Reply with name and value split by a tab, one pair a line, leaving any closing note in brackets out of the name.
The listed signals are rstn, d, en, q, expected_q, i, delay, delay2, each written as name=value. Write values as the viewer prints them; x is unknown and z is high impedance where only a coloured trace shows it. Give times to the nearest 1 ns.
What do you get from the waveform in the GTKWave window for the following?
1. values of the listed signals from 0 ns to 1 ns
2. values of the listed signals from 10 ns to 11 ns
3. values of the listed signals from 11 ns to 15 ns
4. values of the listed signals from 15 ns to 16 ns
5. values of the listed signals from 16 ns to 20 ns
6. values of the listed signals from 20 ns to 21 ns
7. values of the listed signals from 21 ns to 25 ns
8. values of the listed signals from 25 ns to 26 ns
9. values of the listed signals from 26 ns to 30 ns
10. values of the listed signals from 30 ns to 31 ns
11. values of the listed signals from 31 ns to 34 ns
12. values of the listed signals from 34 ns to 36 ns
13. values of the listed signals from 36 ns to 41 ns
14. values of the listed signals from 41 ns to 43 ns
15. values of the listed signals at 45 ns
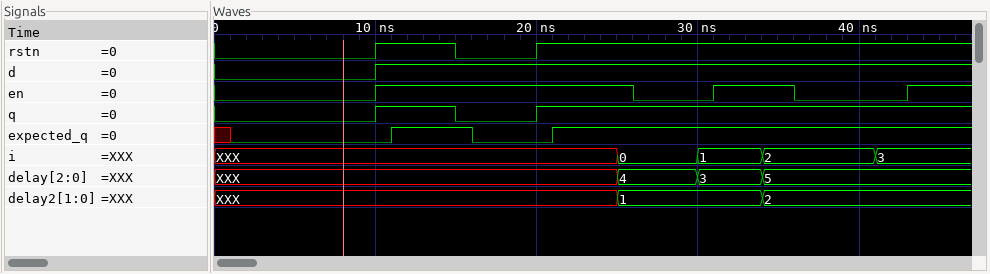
values of the listed signals from 0 ns to 1 ns	rstn=0, d=0, en=0, q=0, expected_q=x, i=XXX, delay=XXX, delay2=XXX
values of the listed signals from 10 ns to 11 ns	rstn=1, d=1, en=1, q=1, expected_q=0, i=XXX, delay=XXX, delay2=XXX
values of the listed signals from 11 ns to 15 ns	rstn=1, d=1, en=1, q=1, expected_q=1, i=XXX, delay=XXX, delay2=XXX
values of the listed signals from 15 ns to 16 ns	rstn=0, d=1, en=1, q=0, expected_q=1, i=XXX, delay=XXX, delay2=XXX
values of the listed signals from 16 ns to 20 ns	rstn=0, d=1, en=1, q=0, expected_q=0, i=XXX, delay=XXX, delay2=XXX
values of the listed signals from 20 ns to 21 ns	rstn=1, d=1, en=1, q=1, expected_q=0, i=XXX, delay=XXX, delay2=XXX
values of the listed signals from 21 ns to 25 ns	rstn=1, d=1, en=1, q=1, expected_q=1, i=XXX, delay=XXX, delay2=XXX
values of the listed signals from 25 ns to 26 ns	rstn=1, d=1, en=1, q=1, expected_q=1, i=0, delay=4, delay2=1
values of the listed signals from 26 ns to 30 ns	rstn=1, d=1, en=0, q=1, expected_q=1, i=0, delay=4, delay2=1
values of the listed signals from 30 ns to 31 ns	rstn=1, d=1, en=0, q=1, expected_q=1, i=1, delay=3, delay2=1
values of the listed signals from 31 ns to 34 ns	rstn=1, d=1, en=1, q=1, expected_q=1, i=1, delay=3, delay2=1
values of the listed signals from 34 ns to 36 ns	rstn=1, d=1, en=1, q=1, expected_q=1, i=2, delay=5, delay2=2
values of the listed signals from 36 ns to 41 ns	rstn=1, d=1, en=0, q=1, expected_q=1, i=2, delay=5, delay2=2
values of the listed signals from 41 ns to 43 ns	rstn=1, d=1, en=0, q=1, expected_q=1, i=3, delay=5, delay2=2
values of the listed signals at 45 ns	rstn=1, d=1, en=1, q=1, expected_q=1, i=3, delay=5, delay2=2
